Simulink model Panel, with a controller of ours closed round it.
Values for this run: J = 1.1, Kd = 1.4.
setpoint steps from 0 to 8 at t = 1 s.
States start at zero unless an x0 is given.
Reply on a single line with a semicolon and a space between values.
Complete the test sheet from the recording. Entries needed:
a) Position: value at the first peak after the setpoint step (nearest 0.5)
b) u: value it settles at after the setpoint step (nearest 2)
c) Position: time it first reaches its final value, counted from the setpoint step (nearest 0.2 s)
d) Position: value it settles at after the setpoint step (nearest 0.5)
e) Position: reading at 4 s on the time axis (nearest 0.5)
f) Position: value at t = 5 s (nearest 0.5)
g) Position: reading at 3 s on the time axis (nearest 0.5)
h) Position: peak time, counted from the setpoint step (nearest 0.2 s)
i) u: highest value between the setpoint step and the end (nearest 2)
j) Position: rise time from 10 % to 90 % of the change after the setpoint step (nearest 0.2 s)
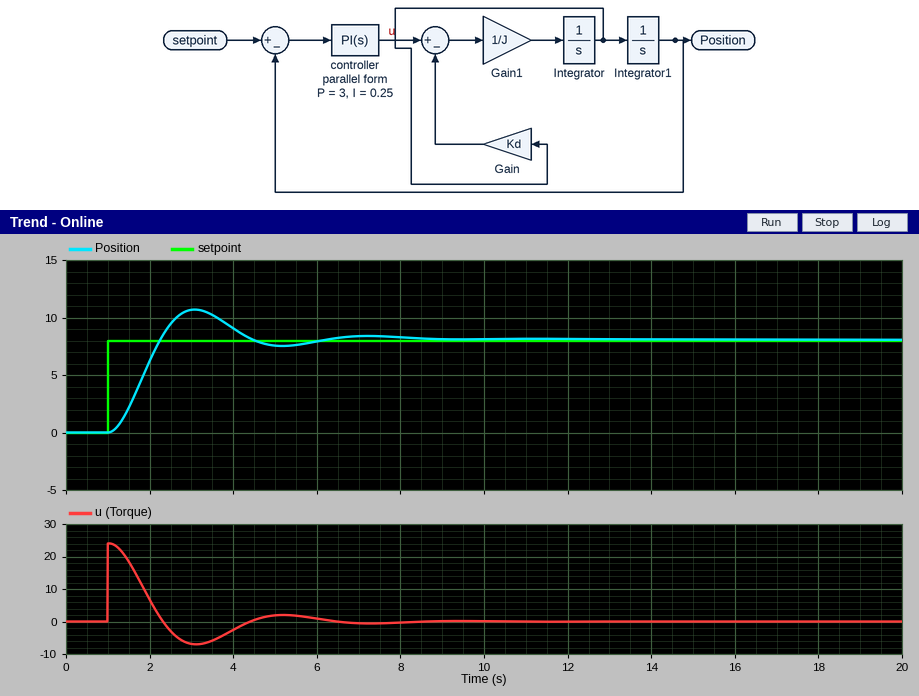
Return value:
10.5; 0; 1.2 s; 8.0; 9.0; 7.5; 10.5; 2.0 s; 24; 0.8 s
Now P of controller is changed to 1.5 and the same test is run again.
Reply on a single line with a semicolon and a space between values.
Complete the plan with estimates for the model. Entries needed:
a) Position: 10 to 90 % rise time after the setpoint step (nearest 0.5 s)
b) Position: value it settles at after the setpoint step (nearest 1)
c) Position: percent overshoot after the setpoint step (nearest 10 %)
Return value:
1.5 s; 8; 30 %
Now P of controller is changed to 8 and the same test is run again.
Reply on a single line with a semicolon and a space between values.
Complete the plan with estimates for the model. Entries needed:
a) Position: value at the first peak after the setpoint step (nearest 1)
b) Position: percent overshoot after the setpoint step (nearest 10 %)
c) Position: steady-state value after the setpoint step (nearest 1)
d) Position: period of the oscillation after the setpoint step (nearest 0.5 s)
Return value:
12; 50 %; 8; 2.5 s
